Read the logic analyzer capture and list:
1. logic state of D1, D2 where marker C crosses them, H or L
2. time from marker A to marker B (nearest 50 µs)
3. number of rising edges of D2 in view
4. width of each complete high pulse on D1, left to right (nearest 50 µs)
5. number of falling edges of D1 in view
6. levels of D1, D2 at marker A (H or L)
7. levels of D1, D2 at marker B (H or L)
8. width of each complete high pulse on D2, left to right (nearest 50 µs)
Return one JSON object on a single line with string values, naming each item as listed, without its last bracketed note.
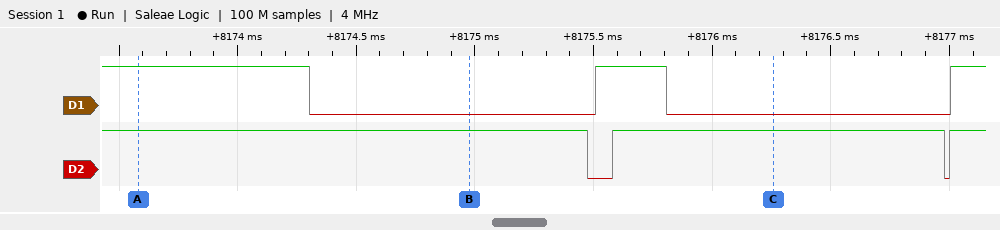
{"logic state of D1, D2 where marker C crosses them, H or L": "D1=L, D2=H", "time from marker A to marker B": "1400 µs", "number of rising edges of D2 in view": "2", "width of each complete high pulse on D1, left to right": "300 µs", "number of falling edges of D1 in view": "2", "levels of D1, D2 at marker A": "D1=H, D2=H", "levels of D1, D2 at marker B": "D1=L, D2=H", "width of each complete high pulse on D2, left to right": "1400 µs"}
